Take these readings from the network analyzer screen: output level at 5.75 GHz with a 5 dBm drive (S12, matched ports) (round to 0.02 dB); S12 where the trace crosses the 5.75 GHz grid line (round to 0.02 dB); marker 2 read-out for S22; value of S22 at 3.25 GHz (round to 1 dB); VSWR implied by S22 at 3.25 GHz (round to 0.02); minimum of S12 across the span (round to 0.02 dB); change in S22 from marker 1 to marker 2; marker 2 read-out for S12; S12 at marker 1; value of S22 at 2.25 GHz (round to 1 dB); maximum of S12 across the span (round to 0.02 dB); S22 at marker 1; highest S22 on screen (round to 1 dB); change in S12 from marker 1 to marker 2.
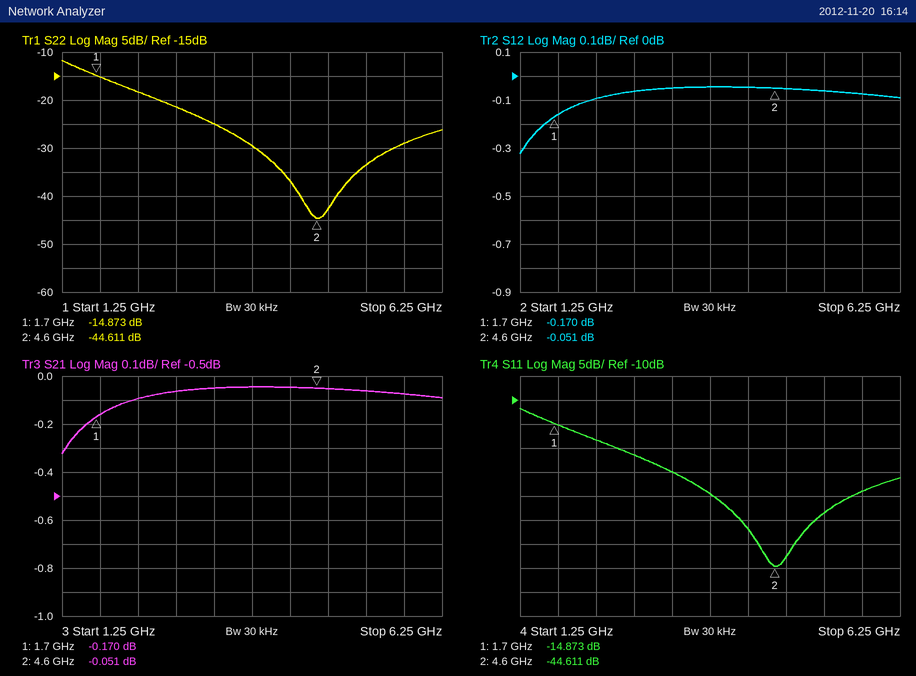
4.92 dBm
-0.08 dB
-44.611 dB
-25 dB
1.12
-0.32 dB
-29.738 dB
-0.051 dB
-0.170 dB
-18 dB
-0.04 dB
-14.873 dB
-12 dB
0.119 dB
